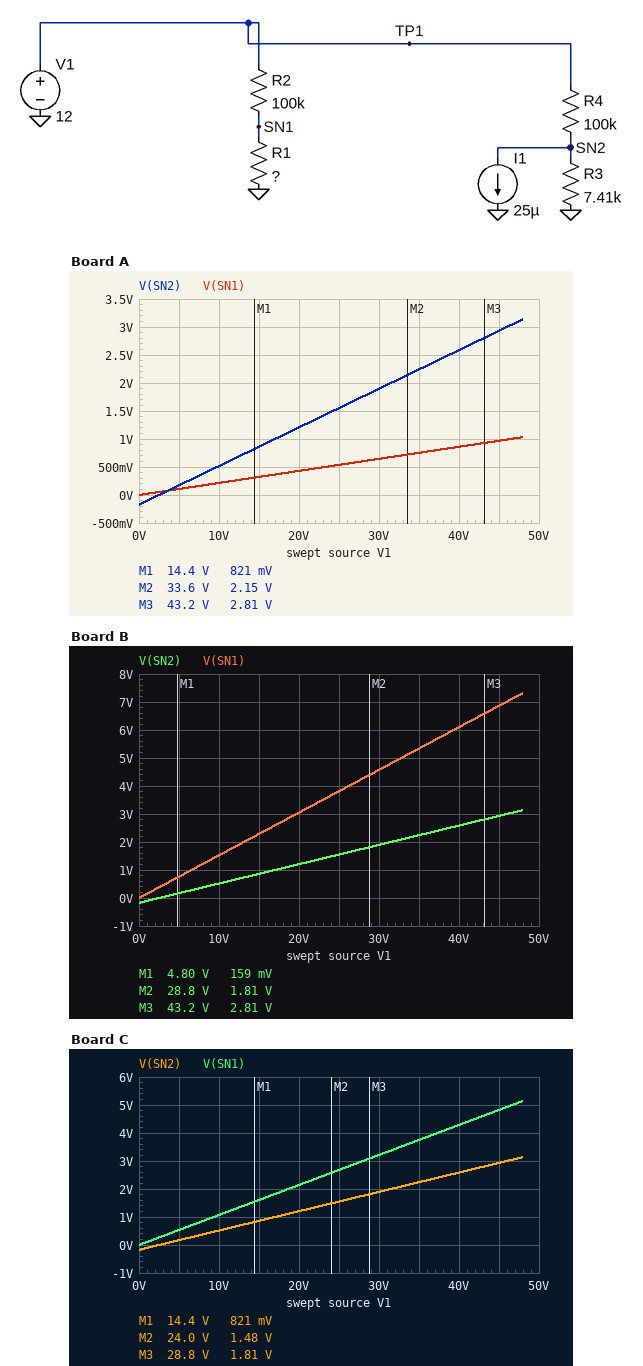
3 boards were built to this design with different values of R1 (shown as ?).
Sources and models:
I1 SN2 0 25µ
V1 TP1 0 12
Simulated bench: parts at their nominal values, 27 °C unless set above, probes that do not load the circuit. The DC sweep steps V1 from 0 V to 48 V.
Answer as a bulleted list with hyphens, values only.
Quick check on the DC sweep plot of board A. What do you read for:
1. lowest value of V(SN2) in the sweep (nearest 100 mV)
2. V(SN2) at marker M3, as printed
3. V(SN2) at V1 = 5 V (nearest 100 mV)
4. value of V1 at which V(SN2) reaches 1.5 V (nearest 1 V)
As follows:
- -200 mV
- 2.81 V
- 200 mV
- 24 V
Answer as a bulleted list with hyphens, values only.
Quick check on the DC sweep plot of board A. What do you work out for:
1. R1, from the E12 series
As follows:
- 2.2 kΩ
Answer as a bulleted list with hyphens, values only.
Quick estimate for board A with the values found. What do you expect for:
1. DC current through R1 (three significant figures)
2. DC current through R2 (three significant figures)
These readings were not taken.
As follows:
- 117 µA
- 117 µA
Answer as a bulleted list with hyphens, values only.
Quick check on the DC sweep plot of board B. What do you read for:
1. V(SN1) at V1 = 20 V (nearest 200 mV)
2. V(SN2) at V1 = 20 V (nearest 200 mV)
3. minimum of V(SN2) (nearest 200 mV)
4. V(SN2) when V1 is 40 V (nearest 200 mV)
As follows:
- 3.0 V
- 1.2 V
- -200 mV
- 2.6 V
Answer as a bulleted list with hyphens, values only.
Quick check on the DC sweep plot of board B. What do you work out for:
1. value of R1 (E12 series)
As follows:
- 18 kΩ
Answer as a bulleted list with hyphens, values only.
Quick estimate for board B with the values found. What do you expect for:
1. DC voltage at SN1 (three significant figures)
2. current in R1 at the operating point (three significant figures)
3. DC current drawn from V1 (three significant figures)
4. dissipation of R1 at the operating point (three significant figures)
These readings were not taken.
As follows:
- 1.83 V
- 102 µA
- 215 µA
- 186 µW
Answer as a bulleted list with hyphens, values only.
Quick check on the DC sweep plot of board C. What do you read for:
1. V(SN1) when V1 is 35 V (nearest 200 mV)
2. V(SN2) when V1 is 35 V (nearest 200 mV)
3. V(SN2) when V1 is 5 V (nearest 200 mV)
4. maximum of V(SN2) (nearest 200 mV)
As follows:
- 3.8 V
- 2.2 V
- 200 mV
- 3.2 V
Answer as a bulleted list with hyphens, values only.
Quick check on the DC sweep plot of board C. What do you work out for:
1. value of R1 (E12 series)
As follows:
- 12 kΩ
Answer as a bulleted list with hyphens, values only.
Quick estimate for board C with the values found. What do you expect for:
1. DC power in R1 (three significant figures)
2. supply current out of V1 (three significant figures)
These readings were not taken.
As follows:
- 138 µW
- 221 µA
